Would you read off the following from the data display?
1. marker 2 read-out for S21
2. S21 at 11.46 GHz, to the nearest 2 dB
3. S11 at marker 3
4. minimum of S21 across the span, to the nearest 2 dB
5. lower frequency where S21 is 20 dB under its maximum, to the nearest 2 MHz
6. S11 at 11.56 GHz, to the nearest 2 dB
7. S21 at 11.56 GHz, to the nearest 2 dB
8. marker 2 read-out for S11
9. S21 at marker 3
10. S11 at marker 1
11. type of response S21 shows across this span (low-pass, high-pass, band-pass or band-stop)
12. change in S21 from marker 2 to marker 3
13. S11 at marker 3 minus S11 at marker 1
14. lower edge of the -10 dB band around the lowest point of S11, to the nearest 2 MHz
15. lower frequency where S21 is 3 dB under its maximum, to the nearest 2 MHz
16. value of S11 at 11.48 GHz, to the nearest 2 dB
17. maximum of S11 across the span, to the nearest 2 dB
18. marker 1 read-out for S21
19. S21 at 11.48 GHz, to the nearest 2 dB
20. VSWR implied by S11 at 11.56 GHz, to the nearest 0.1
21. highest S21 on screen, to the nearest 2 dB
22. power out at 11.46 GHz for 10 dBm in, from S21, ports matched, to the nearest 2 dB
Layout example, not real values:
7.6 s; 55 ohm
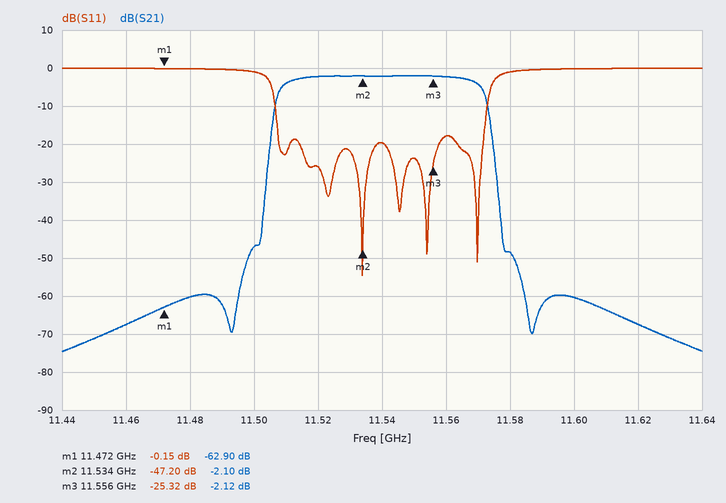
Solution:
-2.10 dB; -68 dB; -25.32 dB; -74 dB; 11.504 GHz; -18 dB; -2 dB; -47.20 dB; -2.12 dB; -0.15 dB; band-pass; -0.02 dB; -25.17 dB; 11.506 GHz; 11.508 GHz; 0 dB; 0 dB; -62.90 dB; -60 dB; 1.3; -2 dB; -58 dBm
